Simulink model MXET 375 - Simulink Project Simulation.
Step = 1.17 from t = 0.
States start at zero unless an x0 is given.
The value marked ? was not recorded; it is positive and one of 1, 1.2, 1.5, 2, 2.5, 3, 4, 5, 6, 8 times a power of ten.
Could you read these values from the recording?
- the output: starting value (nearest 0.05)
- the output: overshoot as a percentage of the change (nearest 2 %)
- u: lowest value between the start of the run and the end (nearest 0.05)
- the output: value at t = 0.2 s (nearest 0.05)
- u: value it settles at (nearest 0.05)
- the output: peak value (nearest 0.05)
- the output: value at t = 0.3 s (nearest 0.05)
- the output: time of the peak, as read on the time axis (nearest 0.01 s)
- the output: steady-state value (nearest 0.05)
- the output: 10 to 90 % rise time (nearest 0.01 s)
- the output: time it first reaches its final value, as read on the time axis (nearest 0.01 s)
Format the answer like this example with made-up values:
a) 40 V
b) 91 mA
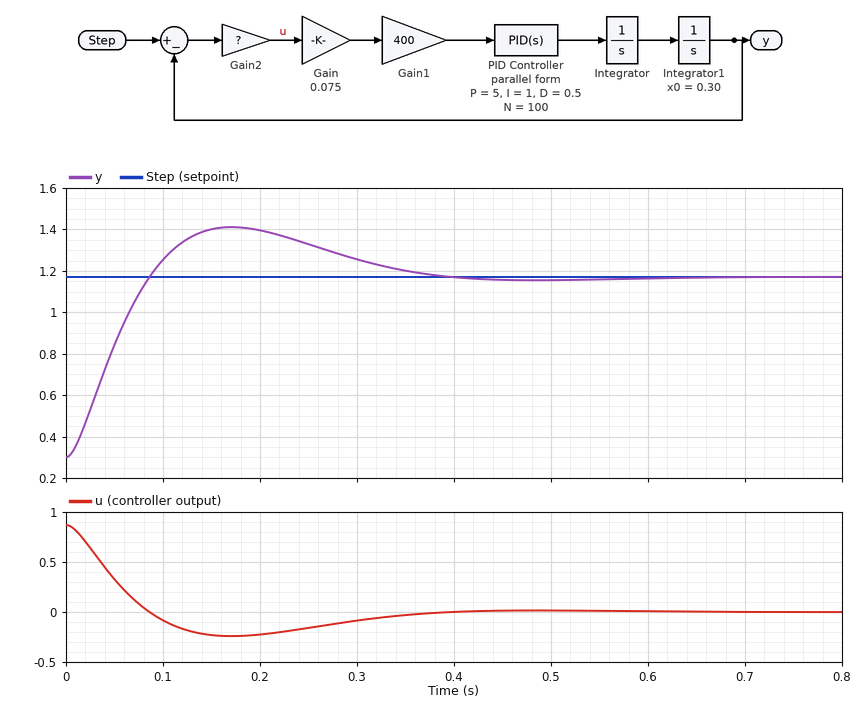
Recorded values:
a) 0.30
b) 28 %
c) -0.25
d) 1.40
e) 0.00
f) 1.40
g) 1.25
h) 0.17 s
i) 1.15
j) 0.06 s
k) 0.09 s
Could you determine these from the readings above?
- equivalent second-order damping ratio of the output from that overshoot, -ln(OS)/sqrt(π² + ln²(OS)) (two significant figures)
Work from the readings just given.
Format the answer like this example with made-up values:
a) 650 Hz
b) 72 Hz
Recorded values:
a) 0.38
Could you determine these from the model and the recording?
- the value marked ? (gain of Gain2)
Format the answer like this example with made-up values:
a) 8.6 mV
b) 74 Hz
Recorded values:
a) 1
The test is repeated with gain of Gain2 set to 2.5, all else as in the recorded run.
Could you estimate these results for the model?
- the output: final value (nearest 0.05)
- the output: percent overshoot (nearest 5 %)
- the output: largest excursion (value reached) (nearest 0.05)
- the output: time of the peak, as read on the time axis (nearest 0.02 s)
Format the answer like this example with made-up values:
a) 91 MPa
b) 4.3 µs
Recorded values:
a) 1.15
b) 20 %
c) 1.35
d) 0.08 s
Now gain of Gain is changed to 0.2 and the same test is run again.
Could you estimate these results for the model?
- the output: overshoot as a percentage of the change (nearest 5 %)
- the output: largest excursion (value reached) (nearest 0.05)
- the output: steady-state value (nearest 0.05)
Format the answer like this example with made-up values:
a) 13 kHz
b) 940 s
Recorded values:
a) 20 %
b) 1.35
c) 1.15
